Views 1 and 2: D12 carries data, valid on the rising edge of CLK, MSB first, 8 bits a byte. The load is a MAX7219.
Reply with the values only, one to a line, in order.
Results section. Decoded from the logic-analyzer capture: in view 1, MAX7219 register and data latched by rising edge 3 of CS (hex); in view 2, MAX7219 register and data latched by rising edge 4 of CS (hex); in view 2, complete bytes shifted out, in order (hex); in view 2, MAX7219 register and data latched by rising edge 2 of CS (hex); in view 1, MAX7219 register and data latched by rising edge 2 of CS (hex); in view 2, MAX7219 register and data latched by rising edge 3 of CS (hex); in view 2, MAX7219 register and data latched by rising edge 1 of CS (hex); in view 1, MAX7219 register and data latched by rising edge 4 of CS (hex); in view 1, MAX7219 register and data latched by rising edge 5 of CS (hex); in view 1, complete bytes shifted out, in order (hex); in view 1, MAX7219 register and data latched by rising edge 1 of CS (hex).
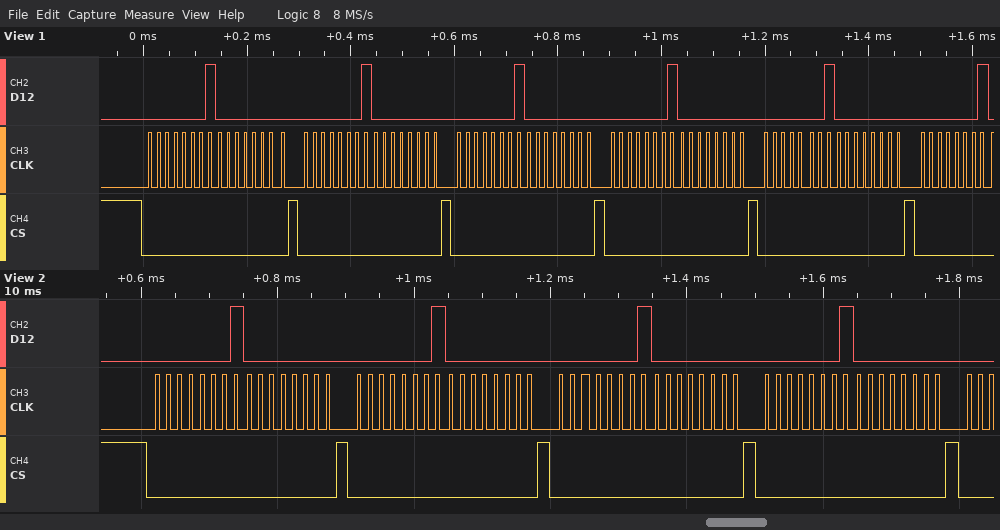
register 0x1, data 0x00
register 0x1, data 0x00
0x01 0x00 0x01 0x00 0x01 0x00 0x01 0x00
register 0x1, data 0x00
register 0x1, data 0x00
register 0x1, data 0x00
register 0x1, data 0x00
register 0x1, data 0x00
register 0x1, data 0x00
01 00 01 00 01 00 01 00 01 00 01
register 0x1, data 0x00
